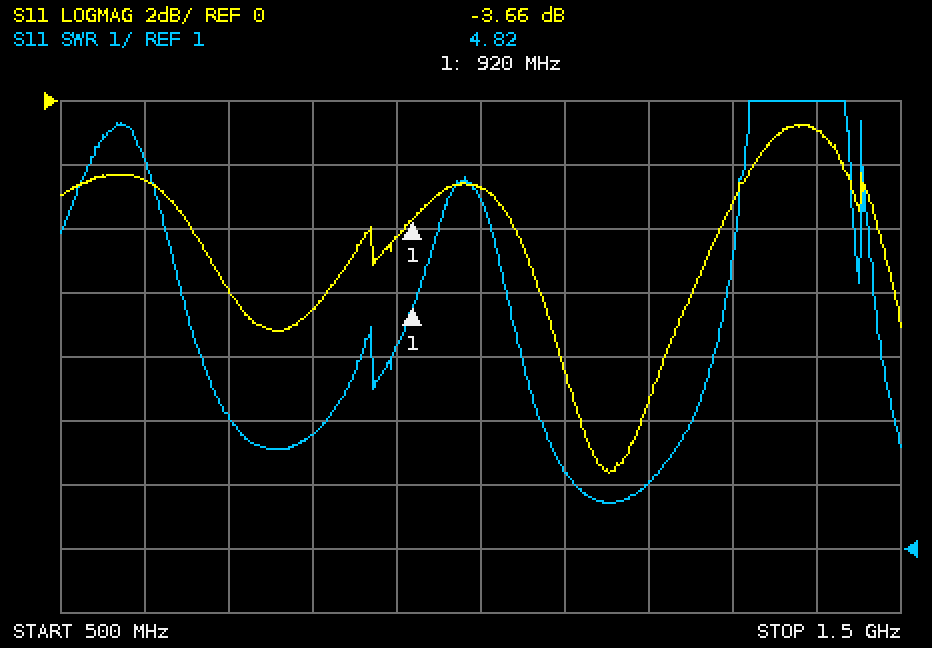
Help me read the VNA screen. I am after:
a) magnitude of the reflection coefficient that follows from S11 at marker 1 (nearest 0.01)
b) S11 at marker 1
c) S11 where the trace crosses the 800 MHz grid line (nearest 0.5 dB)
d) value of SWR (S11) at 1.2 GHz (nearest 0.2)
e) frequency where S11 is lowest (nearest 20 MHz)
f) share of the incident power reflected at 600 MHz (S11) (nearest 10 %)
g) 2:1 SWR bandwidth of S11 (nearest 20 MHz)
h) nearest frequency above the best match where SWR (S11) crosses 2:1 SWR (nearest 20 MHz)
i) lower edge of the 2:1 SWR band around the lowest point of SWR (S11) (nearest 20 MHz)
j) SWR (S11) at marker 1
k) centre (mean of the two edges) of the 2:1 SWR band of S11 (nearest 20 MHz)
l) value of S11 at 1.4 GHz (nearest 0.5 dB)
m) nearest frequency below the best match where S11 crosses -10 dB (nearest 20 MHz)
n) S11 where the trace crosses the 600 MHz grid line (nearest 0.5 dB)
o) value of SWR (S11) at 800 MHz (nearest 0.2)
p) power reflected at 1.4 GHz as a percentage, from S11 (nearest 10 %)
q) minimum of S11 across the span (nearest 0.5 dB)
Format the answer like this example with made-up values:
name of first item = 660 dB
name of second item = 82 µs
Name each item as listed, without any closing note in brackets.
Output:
magnitude of the reflection coefficient that follows from S11 at marker 1 = 0.66
S11 at marker 1 = -3.66 dB
S11 where the trace crosses the 800 MHz grid line = -6.5 dB
value of SWR (S11) at 1.2 GHz = 2.0
frequency where S11 is lowest = 1.16 GHz
share of the incident power reflected at 600 MHz (S11) = 60 %
2:1 SWR bandwidth of S11 = 80 MHz
nearest frequency above the best match where SWR (S11) crosses 2:1 SWR = 1.20 GHz
lower edge of the 2:1 SWR band around the lowest point of SWR (S11) = 1.12 GHz
SWR (S11) at marker 1 = 4.82
centre (mean of the two edges) of the 2:1 SWR band of S11 = 1.16 GHz
value of S11 at 1.4 GHz = -1.0 dB
nearest frequency below the best match where S11 crosses -10 dB = 1.12 GHz
S11 where the trace crosses the 600 MHz grid line = -2.5 dB
value of SWR (S11) at 800 MHz = 2.8
power reflected at 1.4 GHz as a percentage, from S11 = 80 %
minimum of S11 across the span = -11.5 dB
